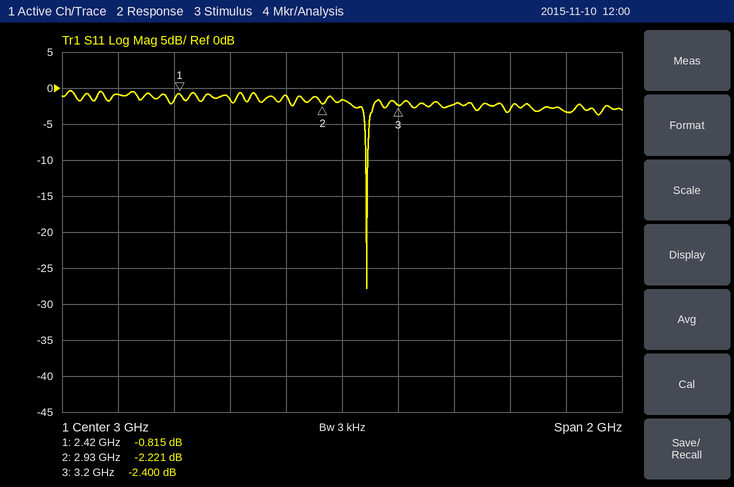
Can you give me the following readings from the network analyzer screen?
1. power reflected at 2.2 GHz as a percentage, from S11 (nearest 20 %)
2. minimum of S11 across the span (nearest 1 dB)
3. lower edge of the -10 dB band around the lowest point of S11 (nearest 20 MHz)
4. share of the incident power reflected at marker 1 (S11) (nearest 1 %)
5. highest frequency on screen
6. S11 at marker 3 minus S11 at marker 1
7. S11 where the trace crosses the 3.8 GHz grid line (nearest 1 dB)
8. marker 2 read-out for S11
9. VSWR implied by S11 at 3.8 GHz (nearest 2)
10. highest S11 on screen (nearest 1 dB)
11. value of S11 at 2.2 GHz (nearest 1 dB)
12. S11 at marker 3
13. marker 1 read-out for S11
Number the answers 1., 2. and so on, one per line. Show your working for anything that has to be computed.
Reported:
1. 10^(-1/10) ≈ 79.4 %, so 80 % to the nearest 20 %
2. -28 dB
3. 3.08 GHz
4. 10^(-0.815/10) ≈ 83 %
5. 4 GHz
6. -2.4 − (-0.815) = -1.585 dB
7. -3 dB
8. -2.221 dB
9. |Γ| = 10^(-3/20) = 0.7079; VSWR = (1 + 0.7079)/(1 − 0.7079) ≈ 6
10. 0 dB
11. -1 dB
12. -2.400 dB
13. -0.815 dB
